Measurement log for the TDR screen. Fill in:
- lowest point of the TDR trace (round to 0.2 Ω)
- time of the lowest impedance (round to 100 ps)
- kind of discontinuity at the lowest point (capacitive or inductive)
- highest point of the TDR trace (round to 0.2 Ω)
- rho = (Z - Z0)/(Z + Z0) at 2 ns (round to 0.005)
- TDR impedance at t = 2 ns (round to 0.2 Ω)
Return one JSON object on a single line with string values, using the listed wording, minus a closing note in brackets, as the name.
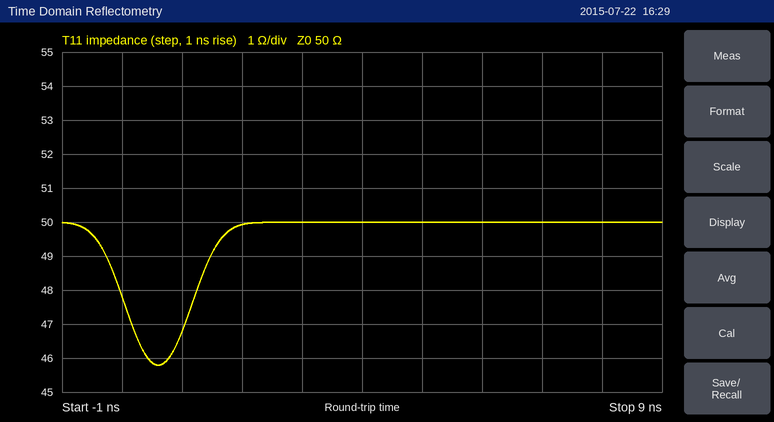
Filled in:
{"lowest point of the TDR trace": "45.8 Ω", "time of the lowest impedance": "600 ps", "kind of discontinuity at the lowest point": "capacitive", "highest point of the TDR trace": "50.0 Ω", "rho = (Z - Z0)/(Z + Z0) at 2 ns": "0.000", "TDR impedance at t = 2 ns": "50.0 Ω"}
